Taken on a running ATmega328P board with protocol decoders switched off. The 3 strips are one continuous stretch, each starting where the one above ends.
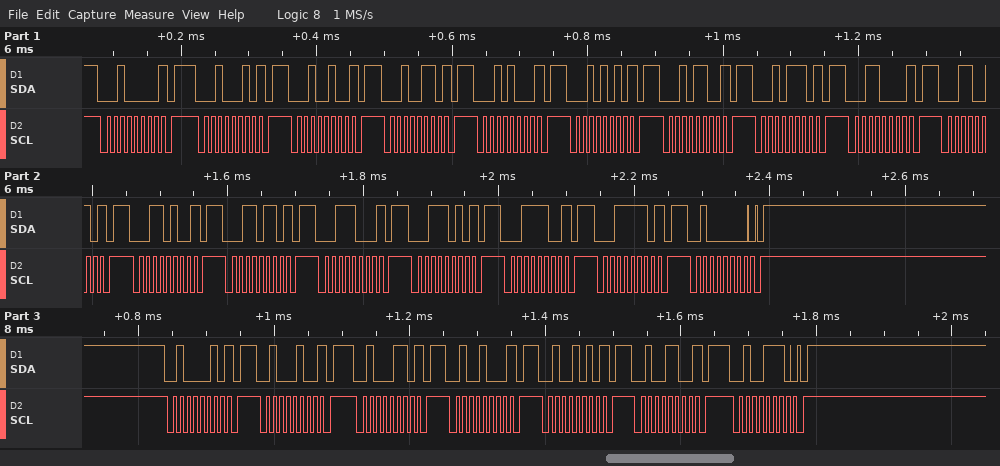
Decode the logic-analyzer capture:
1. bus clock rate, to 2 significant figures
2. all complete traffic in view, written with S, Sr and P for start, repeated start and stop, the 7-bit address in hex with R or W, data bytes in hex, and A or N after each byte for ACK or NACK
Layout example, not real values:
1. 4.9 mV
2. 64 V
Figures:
1. 100 kHz
2. S 10W N P S 11W N P S 12W N P S 13W N P S 14W N P S 15W N P S 16W N P S 17W N P S 18W N P S 19W N P S 1AW N P S 1BW N P S 1CW N P S 1DW N P S 1EW N P S 1FW N P S 20W A P S 21W N P S 22W N P S 23W N P S 24W N P S 25W N P S 26W N P S 27W A P
